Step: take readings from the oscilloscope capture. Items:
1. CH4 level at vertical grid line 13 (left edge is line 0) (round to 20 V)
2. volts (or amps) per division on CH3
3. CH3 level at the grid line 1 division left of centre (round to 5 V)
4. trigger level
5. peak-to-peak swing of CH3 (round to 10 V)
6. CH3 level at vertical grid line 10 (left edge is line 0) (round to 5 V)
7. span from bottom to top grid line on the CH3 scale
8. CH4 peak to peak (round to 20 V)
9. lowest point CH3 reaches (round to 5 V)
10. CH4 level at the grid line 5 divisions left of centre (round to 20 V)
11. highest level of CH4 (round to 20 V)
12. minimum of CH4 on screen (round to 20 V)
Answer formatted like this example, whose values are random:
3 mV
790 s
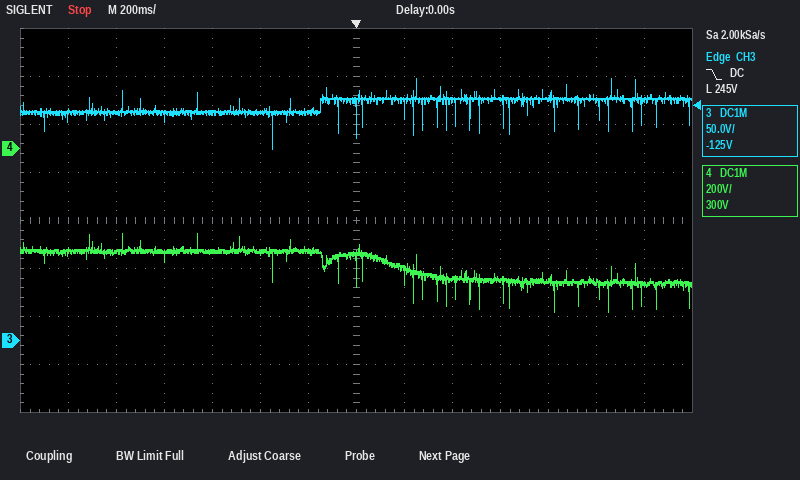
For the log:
-560 V
50 V
240 V
245 V
70 V
250 V
400 V
320 V
200 V
-420 V
-360 V
-680 V
